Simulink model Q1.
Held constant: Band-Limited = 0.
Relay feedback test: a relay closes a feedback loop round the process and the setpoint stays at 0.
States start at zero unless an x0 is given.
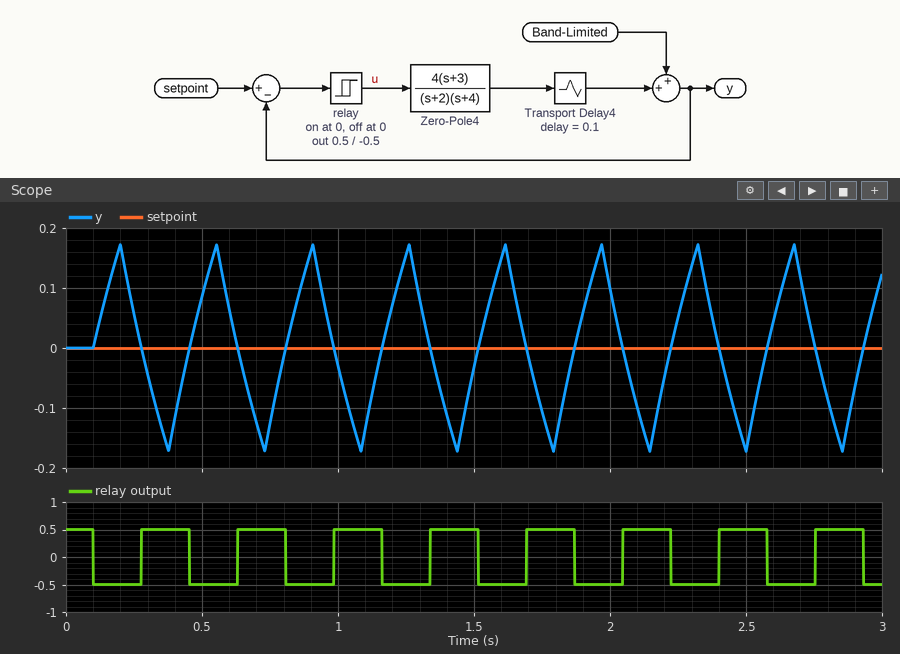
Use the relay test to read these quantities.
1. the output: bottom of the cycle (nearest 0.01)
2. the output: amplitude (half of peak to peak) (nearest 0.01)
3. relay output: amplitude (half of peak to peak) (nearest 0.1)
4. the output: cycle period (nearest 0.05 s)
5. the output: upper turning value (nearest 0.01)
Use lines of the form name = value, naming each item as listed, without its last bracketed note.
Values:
the output: bottom of the cycle = -0.17
the output: amplitude (half of peak to peak) = 0.17
relay output: amplitude (half of peak to peak) = 0.5
the output: cycle period = 0.35 s
the output: upper turning value = 0.17
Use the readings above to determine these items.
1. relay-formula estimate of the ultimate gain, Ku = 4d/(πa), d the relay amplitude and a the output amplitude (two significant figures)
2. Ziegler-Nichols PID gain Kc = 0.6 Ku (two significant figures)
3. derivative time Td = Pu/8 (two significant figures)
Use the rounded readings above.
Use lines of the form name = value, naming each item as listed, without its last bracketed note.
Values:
relay-formula estimate of the ultimate gain, Ku = 4d/(πa), d the relay amplitude and a the output amplitude = 3.7
Ziegler-Nichols PID gain Kc = 0.6 Ku = 2.2
derivative time Td = Pu/8 = 0.044 s
